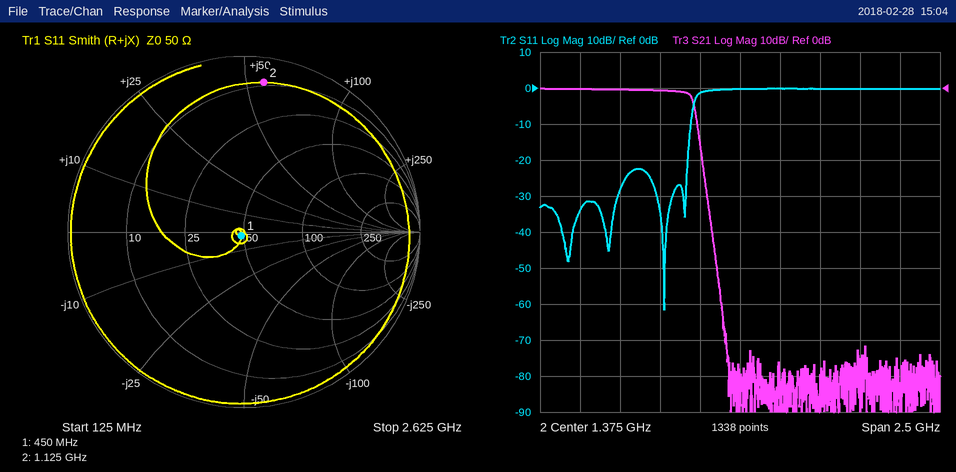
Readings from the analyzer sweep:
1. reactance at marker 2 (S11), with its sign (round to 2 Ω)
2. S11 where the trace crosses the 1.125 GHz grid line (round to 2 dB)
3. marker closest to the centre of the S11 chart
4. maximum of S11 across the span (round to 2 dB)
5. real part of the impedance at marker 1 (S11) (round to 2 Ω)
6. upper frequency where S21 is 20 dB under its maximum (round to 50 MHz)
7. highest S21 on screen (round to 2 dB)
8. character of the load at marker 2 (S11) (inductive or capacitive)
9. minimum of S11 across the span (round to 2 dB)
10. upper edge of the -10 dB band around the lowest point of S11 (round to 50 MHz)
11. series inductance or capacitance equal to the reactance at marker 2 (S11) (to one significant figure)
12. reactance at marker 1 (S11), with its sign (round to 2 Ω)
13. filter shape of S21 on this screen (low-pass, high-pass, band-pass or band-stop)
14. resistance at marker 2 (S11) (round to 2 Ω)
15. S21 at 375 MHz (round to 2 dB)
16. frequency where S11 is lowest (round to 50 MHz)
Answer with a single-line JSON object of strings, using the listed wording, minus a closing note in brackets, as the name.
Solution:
{"reactance at marker 2 (S11), with its sign": "+56 Ω", "S11 where the trace crosses the 1.125 GHz grid line": "-2 dB", "marker closest to the centre of the S11 chart": "marker 1", "maximum of S11 across the span": "0 dB", "real part of the impedance at marker 1 (S11)": "48 Ω", "upper frequency where S21 is 20 dB under its maximum": "1.15 GHz", "highest S21 on screen": "0 dB", "character of the load at marker 2 (S11)": "inductive", "minimum of S11 across the span": "-62 dB", "upper edge of the -10 dB band around the lowest point of S11": "1.05 GHz", "series inductance or capacitance equal to the reactance at marker 2 (S11)": "8 nH", "reactance at marker 1 (S11), with its sign": "-2 Ω", "filter shape of S21 on this screen": "low-pass", "resistance at marker 2 (S11)": "8 Ω", "S21 at 375 MHz": "0 dB", "frequency where S11 is lowest": "900 MHz"}
